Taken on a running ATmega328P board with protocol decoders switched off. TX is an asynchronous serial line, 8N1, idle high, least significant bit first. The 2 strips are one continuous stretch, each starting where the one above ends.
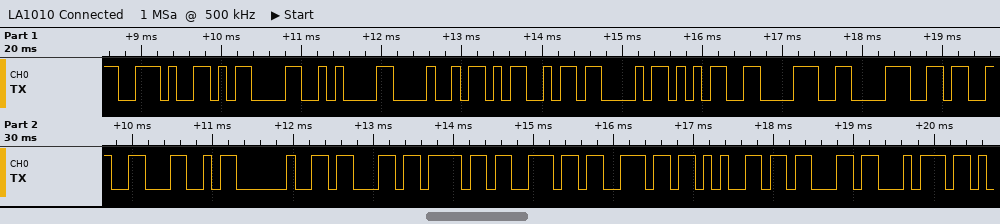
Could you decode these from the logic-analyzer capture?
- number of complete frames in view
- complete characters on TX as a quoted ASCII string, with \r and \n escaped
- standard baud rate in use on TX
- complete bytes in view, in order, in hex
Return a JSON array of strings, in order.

["19", "\".\\r\\nHMC5883L connect\"", "9600 baud", "2E 0D 0A 48 4D 43 35 38 38 33 4C 20 63 6F 6E 6E 65 63 74"]
